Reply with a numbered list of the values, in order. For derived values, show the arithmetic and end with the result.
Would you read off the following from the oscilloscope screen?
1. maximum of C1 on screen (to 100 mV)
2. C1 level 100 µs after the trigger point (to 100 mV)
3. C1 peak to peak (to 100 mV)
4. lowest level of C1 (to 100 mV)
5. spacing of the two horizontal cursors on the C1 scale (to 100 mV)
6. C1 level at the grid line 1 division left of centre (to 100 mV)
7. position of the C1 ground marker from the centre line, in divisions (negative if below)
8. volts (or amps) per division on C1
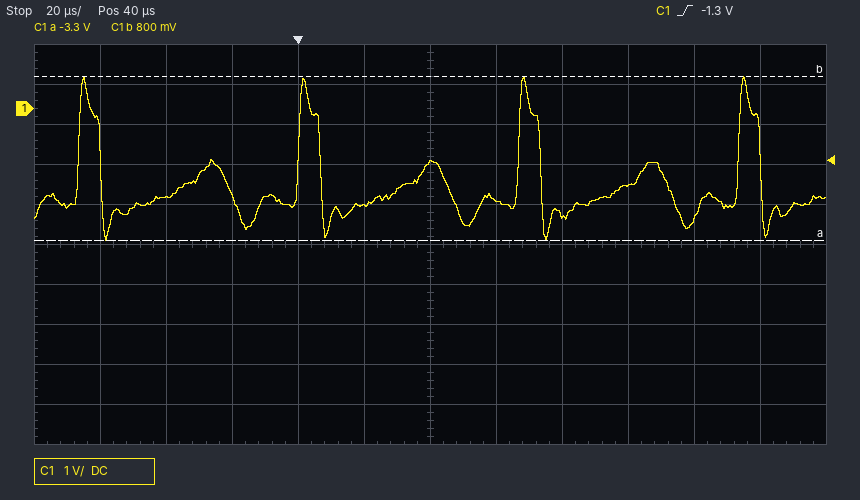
1. 800 mV
2. -1.9 V
3. 800 mV − (-3.3 V) = 4.1 V
4. -3.3 V
5. 4.1 V
6. -2.4 V
7. +3.4 div
8. 1 V
